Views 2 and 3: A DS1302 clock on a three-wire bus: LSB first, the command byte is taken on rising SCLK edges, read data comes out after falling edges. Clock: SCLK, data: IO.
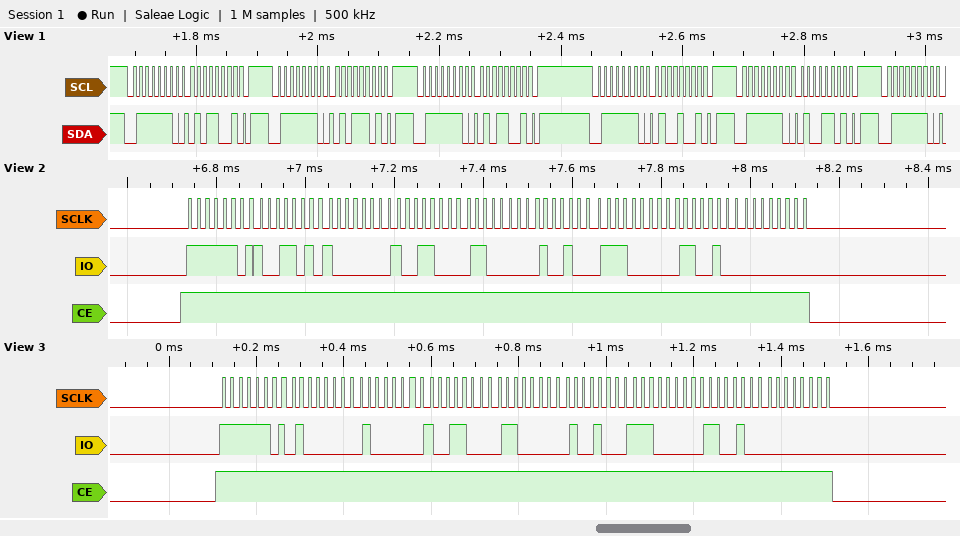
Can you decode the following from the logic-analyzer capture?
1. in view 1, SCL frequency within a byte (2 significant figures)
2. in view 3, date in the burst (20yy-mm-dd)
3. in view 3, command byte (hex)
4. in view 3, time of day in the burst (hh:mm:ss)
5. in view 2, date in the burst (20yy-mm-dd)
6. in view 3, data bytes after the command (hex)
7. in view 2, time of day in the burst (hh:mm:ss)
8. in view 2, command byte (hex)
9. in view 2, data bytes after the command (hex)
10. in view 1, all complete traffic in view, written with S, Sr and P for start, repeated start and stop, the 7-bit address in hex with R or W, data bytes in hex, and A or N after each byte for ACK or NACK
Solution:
100 kHz
2026-12-06
0xBF
19:02:02
2026-12-06
02 02 19 06 12 07 26 00
19:01:59
0xBF
59 01 19 06 12 07 26 00
S 3FW A 59 A P S 3FW A 5D A P S 3FW A 59 A P S 3FW A 49 A P S 3FW A 4D A P S 3FW A
